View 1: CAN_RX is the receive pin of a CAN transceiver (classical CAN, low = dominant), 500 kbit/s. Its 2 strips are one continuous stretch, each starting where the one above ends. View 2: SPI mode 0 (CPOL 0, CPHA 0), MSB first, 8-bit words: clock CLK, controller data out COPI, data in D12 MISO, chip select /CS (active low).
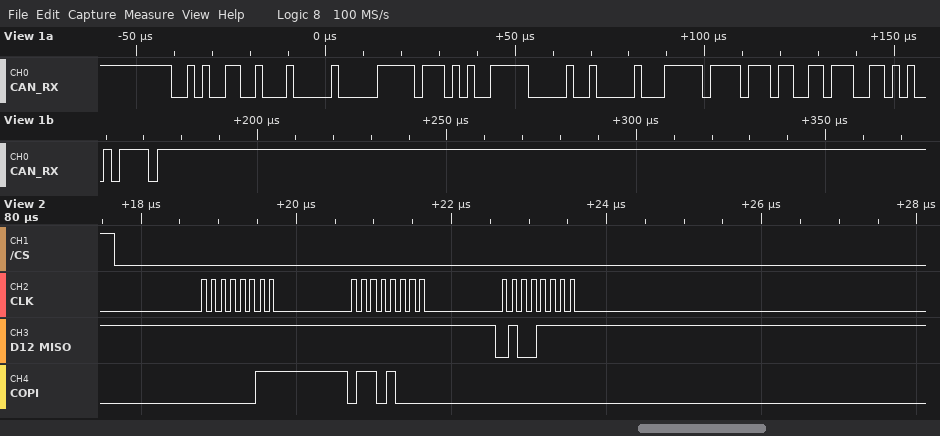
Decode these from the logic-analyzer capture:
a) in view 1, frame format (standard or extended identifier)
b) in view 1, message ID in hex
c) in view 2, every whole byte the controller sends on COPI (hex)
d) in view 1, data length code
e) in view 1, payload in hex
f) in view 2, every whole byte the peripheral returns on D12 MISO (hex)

standard
0x299
0x03 0x68 0x00
8
01 FD 4F 81 00 FF BB 37
0xFF 0xFF 0x4F
